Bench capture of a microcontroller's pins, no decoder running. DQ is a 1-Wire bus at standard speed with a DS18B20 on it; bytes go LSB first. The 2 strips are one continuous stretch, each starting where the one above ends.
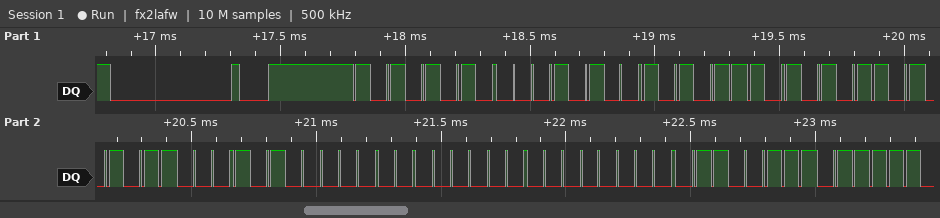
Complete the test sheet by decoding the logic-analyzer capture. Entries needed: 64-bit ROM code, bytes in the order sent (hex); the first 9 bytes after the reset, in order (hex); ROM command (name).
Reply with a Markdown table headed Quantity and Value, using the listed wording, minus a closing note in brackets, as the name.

| Quantity | Value |
|---|---|
| 64-bit ROM code, bytes in the order sent | 28 75 B5 1A 05 00 00 E6 |
| the first 9 bytes after the reset, in order | 55 28 75 B5 1A 05 00 00 E6 |
| ROM command | Match ROM |
